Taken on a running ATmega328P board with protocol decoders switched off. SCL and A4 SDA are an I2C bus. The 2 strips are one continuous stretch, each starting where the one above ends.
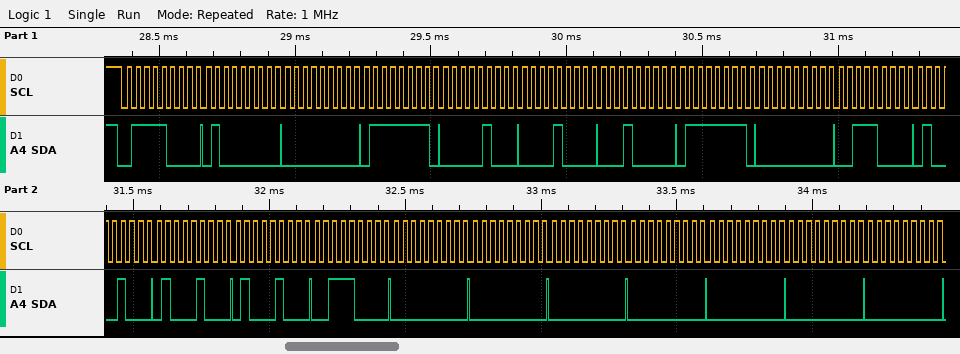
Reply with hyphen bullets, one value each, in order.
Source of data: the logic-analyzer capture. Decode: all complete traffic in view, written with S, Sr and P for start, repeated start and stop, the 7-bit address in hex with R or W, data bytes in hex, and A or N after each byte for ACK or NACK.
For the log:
- S 3CW A 40 A 00 A 7F A 04 A 08 A 10 A 7F A 00 A 38 A 44 A 44 A 44 A 38 A 00 A 00 A 00 A 00 A 00 A 00 A 00 A
